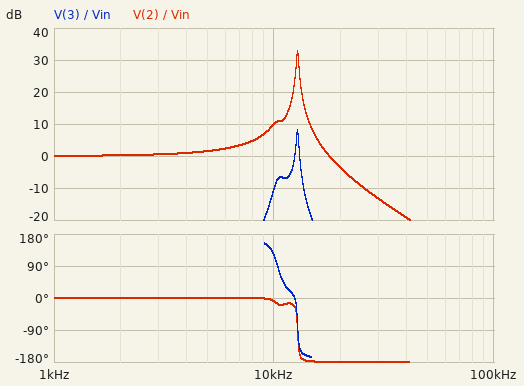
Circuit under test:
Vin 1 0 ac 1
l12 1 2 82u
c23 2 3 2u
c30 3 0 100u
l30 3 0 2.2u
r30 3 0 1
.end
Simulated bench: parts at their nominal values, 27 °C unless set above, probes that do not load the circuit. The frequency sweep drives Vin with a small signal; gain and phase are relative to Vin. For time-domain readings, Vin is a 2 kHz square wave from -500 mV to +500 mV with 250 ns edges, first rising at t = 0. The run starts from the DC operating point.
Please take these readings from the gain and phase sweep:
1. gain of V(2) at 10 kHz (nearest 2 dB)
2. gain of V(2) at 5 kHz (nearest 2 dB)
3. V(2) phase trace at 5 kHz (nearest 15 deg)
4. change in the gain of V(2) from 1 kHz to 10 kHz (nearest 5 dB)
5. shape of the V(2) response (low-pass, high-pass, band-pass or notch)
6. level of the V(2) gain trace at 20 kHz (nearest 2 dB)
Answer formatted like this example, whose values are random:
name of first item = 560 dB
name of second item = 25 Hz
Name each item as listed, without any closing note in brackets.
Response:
gain of V(2) at 10 kHz = 10 dB
gain of V(2) at 5 kHz = 2 dB
V(2) phase trace at 5 kHz = 0 deg
change in the gain of V(2) from 1 kHz to 10 kHz = 10 dB
shape of the V(2) response = low-pass
level of the V(2) gain trace at 20 kHz = -4 dB
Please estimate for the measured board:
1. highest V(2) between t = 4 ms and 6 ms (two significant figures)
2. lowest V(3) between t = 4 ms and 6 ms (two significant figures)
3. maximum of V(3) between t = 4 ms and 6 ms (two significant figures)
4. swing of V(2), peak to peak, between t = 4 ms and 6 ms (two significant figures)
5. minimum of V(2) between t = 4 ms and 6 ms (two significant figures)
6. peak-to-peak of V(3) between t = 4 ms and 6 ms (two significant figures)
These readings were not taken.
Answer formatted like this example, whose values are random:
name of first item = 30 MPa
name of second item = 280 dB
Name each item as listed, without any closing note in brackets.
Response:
highest V(2) between t = 4 ms and 6 ms = 1.2 V
lowest V(3) between t = 4 ms and 6 ms = -57 mV
maximum of V(3) between t = 4 ms and 6 ms = 57 mV
swing of V(2), peak to peak, between t = 4 ms and 6 ms = 2.4 V
minimum of V(2) between t = 4 ms and 6 ms = -1.2 V
peak-to-peak of V(3) between t = 4 ms and 6 ms = 110 mV
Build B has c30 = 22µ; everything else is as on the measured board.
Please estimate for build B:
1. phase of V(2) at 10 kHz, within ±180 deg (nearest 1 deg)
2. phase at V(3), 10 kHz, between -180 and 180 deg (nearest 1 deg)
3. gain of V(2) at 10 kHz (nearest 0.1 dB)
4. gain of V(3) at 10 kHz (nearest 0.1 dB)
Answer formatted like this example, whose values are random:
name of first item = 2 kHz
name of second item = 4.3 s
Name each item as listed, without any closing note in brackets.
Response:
phase of V(2) at 10 kHz, within ±180 deg = 0 deg
phase at V(3), 10 kHz, between -180 and 180 deg = 170 deg
gain of V(2) at 10 kHz = 9.4 dB
gain of V(3) at 10 kHz = -23.9 dB
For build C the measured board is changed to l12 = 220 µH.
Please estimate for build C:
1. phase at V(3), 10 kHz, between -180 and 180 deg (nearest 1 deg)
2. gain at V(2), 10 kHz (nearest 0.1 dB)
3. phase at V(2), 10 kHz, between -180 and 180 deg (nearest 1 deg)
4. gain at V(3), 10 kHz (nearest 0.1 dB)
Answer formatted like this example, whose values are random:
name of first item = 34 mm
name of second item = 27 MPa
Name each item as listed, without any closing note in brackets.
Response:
phase at V(3), 10 kHz, between -180 and 180 deg = -42 deg
gain at V(2), 10 kHz = 1.4 dB
phase at V(2), 10 kHz, between -180 and 180 deg = -171 deg
gain at V(3), 10 kHz = -18.9 dB
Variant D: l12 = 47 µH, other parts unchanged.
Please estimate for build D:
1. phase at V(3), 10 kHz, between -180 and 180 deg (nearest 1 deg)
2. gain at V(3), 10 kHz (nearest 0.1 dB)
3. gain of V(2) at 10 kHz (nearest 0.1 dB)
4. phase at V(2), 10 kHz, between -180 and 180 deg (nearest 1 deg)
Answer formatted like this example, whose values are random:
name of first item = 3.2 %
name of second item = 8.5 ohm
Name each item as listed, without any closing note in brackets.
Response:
phase at V(3), 10 kHz, between -180 and 180 deg = 127 deg
gain at V(3), 10 kHz = -15.9 dB
gain of V(2) at 10 kHz = 4.3 dB
phase at V(2), 10 kHz, between -180 and 180 deg = -3 deg
